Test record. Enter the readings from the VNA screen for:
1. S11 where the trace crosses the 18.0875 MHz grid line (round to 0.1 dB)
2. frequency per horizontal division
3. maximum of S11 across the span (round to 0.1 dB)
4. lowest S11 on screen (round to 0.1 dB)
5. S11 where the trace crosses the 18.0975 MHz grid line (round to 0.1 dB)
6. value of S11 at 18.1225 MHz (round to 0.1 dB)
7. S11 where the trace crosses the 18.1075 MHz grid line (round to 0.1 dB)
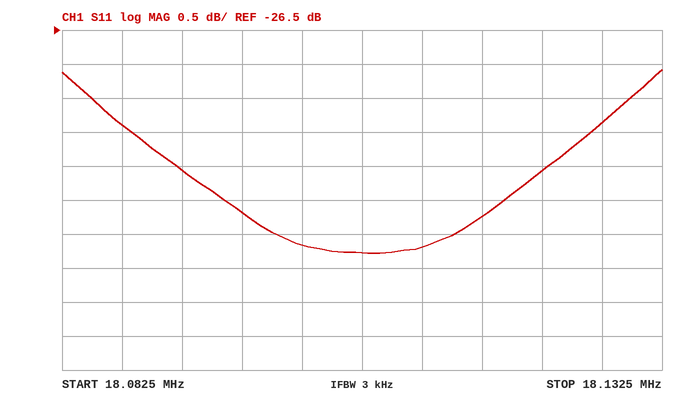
-27.9 dB
5 kHz
-27.1 dB
-29.8 dB
-29.2 dB
-28.6 dB
-29.8 dB
